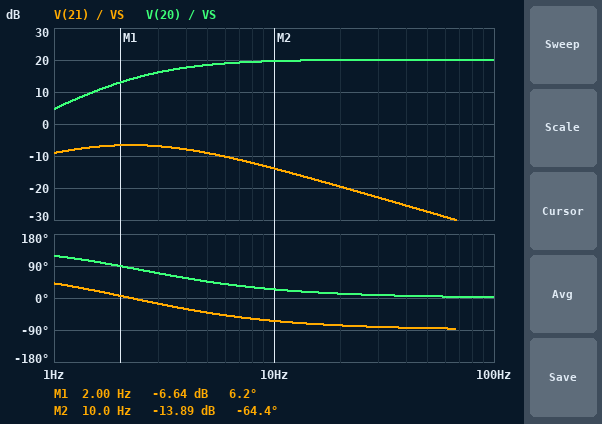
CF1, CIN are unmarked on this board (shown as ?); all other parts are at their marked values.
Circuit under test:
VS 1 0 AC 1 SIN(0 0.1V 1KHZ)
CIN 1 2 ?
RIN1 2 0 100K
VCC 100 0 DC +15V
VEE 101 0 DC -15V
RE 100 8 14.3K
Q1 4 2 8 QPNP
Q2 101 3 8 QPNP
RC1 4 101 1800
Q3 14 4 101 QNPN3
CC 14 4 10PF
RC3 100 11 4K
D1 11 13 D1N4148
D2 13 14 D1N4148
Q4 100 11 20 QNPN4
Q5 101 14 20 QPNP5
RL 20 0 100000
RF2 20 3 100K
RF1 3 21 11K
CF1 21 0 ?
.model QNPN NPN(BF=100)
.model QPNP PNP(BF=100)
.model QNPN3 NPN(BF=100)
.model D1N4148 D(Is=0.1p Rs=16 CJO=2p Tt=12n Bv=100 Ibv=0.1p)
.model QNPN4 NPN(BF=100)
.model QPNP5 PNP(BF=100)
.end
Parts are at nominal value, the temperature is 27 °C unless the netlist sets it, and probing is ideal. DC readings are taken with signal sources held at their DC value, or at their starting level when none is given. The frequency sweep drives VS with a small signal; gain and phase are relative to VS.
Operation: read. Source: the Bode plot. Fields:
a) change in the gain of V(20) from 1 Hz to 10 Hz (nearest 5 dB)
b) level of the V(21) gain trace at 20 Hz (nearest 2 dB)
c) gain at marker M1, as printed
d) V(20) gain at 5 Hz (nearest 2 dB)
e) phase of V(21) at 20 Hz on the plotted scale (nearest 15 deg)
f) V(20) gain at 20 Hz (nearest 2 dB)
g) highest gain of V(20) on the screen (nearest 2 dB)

15 dB
-20 dB
-6.64 dB
18 dB
-75 deg
20 dB
20 dB
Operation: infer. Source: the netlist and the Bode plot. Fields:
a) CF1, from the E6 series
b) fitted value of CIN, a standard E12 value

6.8 µF
680 nF
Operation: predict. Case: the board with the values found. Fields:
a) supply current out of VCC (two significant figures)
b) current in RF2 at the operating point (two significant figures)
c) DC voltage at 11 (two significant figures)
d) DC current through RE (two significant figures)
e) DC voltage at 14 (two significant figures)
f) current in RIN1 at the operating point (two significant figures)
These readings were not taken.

4.6 mA
4.7 µA
700 mV
960 µA
-670 mV
4.8 µA
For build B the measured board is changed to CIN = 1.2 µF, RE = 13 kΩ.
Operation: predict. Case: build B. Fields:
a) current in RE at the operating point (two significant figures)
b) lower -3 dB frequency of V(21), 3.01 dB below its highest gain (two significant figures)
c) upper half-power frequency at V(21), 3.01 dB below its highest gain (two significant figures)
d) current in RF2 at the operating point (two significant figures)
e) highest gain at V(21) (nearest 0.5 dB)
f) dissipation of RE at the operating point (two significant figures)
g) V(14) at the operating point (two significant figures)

1.1 mA
680 mHz
4.2 Hz
5.6 µA
-4.5 dB
15 mW
-770 mV
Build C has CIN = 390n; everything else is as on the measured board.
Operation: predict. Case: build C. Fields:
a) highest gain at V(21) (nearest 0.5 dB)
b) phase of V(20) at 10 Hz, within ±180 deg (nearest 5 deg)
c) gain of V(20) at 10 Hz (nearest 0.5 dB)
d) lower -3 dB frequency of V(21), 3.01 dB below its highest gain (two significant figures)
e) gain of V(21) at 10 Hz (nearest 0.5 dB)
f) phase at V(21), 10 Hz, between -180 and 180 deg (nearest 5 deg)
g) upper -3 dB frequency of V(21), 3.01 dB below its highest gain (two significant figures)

-9.5 dB
35 deg
19.0 dB
1.2 Hz
-14.5 dB
-55 deg
7.5 Hz
